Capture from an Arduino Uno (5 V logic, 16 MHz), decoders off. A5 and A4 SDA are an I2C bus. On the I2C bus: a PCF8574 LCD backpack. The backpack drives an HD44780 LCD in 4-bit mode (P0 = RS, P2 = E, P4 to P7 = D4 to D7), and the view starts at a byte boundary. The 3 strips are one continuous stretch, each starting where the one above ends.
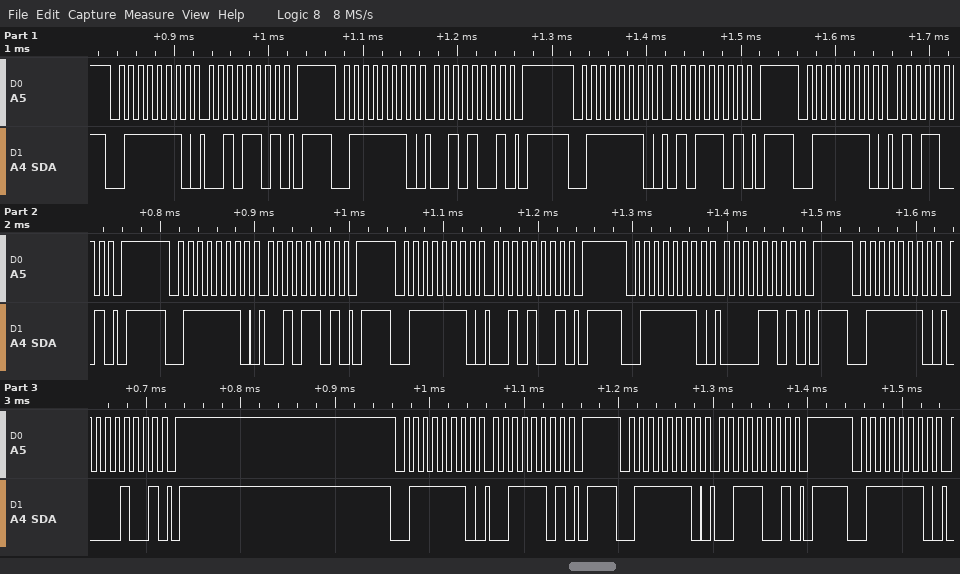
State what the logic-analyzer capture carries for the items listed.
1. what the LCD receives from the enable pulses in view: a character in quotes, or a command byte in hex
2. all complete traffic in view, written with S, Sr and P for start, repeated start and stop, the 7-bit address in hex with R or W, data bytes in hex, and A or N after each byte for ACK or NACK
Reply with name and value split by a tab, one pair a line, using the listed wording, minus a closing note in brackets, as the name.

what the LCD receives from the enable pulses in view: a character in quotes, or a command byte in hex	'%' ' '
all complete traffic in view, written with S, Sr and P for start, repeated start and stop, the 7-bit address in hex with R or W, data bytes in hex, and A or N after each byte for ACK or NACK	S 3FW A 2D A P S 3FW A 29 A P S 3FW A 5D A P S 3FW A 59 A P S 3FW A 2D A P S 3FW A 29 A P S 3FW A 0D A P S 3FW A 09 A P S 3FW A 3D A P S 3FW A 39 A P S 3FW A
